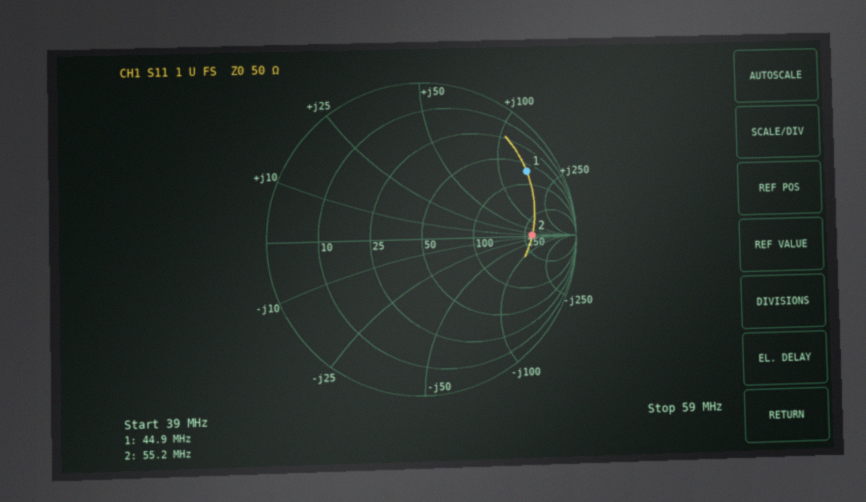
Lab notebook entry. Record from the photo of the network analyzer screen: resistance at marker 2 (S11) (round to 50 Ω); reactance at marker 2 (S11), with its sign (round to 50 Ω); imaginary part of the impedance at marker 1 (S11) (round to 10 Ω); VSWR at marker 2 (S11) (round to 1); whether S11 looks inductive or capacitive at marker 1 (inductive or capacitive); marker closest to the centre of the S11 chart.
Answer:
300 Ω
0 Ω
+150 Ω
6
inductive
marker 2
